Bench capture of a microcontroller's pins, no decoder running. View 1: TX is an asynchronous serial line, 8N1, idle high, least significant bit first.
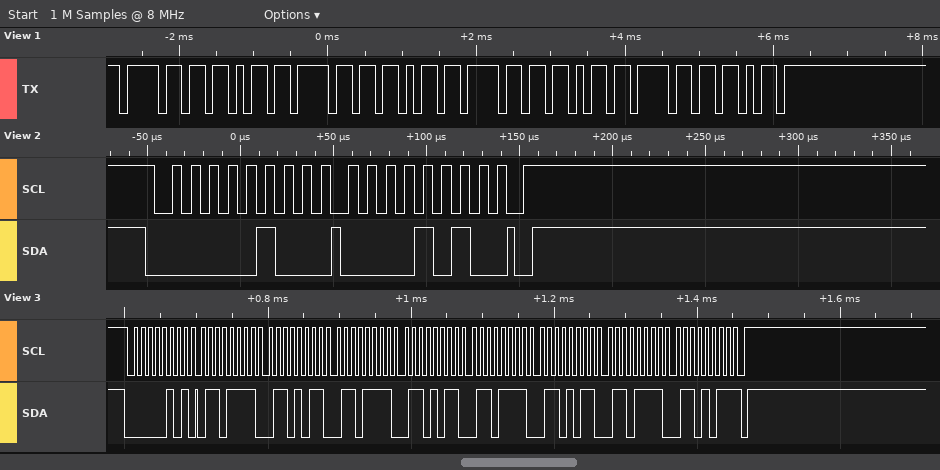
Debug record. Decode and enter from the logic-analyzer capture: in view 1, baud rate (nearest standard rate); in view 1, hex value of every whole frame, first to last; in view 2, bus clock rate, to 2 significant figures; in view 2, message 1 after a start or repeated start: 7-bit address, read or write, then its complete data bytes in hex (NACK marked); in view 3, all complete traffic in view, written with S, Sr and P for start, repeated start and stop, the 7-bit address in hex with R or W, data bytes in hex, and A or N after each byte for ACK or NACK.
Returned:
9600 baud
6F 6B 6F 6B 6F 6B 6F 6B
100 kHz
0x02 write: 0A
S 02R A 6F A 6B A 6F A 6B A 6F A 6B A 6F A 6B N P
